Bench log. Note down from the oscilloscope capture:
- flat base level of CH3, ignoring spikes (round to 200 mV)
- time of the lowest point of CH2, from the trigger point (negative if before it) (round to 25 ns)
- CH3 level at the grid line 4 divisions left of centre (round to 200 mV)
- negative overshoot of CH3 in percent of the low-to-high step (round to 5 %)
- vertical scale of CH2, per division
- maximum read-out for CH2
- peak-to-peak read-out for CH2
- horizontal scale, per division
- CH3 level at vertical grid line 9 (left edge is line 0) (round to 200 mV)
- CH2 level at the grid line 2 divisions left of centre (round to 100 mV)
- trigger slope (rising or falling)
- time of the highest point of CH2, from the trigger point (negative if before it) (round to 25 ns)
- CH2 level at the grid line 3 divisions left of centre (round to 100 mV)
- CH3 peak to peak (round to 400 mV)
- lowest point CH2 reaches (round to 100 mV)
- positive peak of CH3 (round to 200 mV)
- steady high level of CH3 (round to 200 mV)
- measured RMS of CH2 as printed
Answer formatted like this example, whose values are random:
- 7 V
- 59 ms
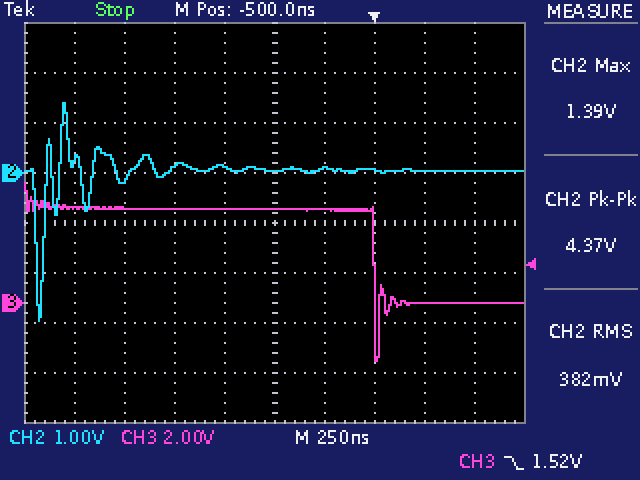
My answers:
- 0.0 V
- -1.675 µs
- 3.8 V
- 60 %
- 1 V
- 1.39 V
- 4.37 V
- 250 ns
- 0.0 V
- 100 mV
- falling
- -1.550 µs
- -100 mV
- 7.2 V
- -3.0 V
- 4.8 V
- 3.8 V
- 382 mV
